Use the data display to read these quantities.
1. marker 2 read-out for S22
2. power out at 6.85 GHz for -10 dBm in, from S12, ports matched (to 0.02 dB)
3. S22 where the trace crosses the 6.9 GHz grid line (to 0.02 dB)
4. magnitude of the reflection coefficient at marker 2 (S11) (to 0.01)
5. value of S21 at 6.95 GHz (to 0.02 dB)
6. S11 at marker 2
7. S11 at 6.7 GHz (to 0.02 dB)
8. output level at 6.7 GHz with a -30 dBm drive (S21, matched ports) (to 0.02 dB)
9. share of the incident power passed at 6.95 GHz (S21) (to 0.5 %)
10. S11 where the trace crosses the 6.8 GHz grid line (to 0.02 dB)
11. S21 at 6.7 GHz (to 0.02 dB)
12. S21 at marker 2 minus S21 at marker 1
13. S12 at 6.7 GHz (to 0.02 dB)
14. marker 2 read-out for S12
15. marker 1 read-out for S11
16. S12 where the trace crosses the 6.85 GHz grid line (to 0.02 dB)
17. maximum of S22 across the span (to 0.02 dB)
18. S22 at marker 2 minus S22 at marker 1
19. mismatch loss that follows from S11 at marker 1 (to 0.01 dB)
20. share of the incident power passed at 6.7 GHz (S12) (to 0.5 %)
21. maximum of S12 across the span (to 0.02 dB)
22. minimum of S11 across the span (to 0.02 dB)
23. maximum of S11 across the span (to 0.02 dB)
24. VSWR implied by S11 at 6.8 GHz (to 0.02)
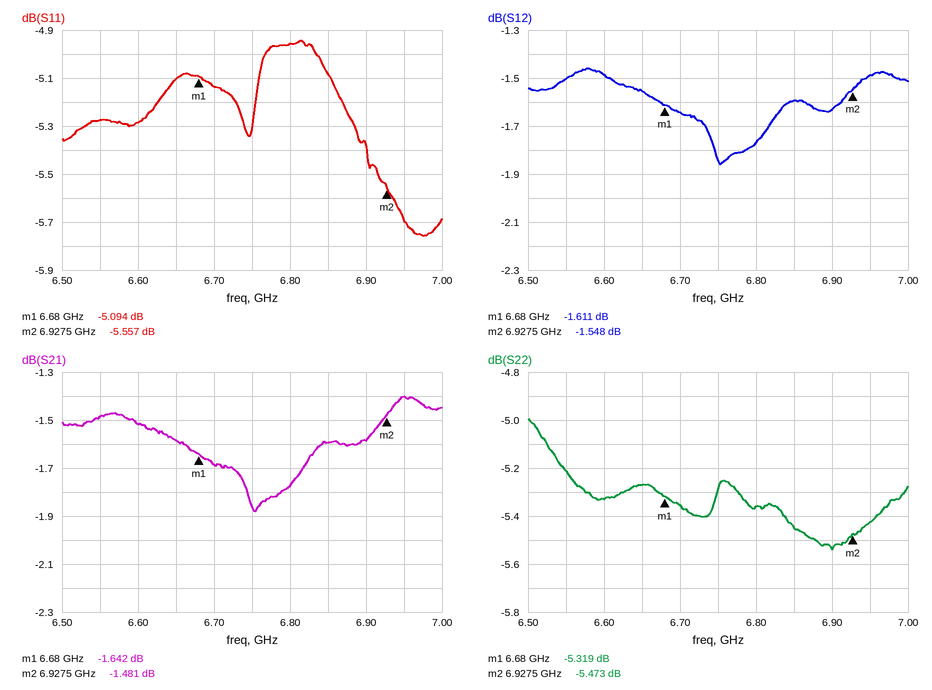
-5.473 dB
-11.60 dBm
-5.54 dB
0.53
-1.40 dB
-5.557 dB
-5.14 dB
-31.68 dBm
72.5 %
-4.96 dB
-1.68 dB
0.161 dB
-1.64 dB
-1.548 dB
-5.094 dB
-1.60 dB
-5.00 dB
-0.154 dB
1.61 dB
68.5 %
-1.46 dB
-5.76 dB
-4.94 dB
3.60
